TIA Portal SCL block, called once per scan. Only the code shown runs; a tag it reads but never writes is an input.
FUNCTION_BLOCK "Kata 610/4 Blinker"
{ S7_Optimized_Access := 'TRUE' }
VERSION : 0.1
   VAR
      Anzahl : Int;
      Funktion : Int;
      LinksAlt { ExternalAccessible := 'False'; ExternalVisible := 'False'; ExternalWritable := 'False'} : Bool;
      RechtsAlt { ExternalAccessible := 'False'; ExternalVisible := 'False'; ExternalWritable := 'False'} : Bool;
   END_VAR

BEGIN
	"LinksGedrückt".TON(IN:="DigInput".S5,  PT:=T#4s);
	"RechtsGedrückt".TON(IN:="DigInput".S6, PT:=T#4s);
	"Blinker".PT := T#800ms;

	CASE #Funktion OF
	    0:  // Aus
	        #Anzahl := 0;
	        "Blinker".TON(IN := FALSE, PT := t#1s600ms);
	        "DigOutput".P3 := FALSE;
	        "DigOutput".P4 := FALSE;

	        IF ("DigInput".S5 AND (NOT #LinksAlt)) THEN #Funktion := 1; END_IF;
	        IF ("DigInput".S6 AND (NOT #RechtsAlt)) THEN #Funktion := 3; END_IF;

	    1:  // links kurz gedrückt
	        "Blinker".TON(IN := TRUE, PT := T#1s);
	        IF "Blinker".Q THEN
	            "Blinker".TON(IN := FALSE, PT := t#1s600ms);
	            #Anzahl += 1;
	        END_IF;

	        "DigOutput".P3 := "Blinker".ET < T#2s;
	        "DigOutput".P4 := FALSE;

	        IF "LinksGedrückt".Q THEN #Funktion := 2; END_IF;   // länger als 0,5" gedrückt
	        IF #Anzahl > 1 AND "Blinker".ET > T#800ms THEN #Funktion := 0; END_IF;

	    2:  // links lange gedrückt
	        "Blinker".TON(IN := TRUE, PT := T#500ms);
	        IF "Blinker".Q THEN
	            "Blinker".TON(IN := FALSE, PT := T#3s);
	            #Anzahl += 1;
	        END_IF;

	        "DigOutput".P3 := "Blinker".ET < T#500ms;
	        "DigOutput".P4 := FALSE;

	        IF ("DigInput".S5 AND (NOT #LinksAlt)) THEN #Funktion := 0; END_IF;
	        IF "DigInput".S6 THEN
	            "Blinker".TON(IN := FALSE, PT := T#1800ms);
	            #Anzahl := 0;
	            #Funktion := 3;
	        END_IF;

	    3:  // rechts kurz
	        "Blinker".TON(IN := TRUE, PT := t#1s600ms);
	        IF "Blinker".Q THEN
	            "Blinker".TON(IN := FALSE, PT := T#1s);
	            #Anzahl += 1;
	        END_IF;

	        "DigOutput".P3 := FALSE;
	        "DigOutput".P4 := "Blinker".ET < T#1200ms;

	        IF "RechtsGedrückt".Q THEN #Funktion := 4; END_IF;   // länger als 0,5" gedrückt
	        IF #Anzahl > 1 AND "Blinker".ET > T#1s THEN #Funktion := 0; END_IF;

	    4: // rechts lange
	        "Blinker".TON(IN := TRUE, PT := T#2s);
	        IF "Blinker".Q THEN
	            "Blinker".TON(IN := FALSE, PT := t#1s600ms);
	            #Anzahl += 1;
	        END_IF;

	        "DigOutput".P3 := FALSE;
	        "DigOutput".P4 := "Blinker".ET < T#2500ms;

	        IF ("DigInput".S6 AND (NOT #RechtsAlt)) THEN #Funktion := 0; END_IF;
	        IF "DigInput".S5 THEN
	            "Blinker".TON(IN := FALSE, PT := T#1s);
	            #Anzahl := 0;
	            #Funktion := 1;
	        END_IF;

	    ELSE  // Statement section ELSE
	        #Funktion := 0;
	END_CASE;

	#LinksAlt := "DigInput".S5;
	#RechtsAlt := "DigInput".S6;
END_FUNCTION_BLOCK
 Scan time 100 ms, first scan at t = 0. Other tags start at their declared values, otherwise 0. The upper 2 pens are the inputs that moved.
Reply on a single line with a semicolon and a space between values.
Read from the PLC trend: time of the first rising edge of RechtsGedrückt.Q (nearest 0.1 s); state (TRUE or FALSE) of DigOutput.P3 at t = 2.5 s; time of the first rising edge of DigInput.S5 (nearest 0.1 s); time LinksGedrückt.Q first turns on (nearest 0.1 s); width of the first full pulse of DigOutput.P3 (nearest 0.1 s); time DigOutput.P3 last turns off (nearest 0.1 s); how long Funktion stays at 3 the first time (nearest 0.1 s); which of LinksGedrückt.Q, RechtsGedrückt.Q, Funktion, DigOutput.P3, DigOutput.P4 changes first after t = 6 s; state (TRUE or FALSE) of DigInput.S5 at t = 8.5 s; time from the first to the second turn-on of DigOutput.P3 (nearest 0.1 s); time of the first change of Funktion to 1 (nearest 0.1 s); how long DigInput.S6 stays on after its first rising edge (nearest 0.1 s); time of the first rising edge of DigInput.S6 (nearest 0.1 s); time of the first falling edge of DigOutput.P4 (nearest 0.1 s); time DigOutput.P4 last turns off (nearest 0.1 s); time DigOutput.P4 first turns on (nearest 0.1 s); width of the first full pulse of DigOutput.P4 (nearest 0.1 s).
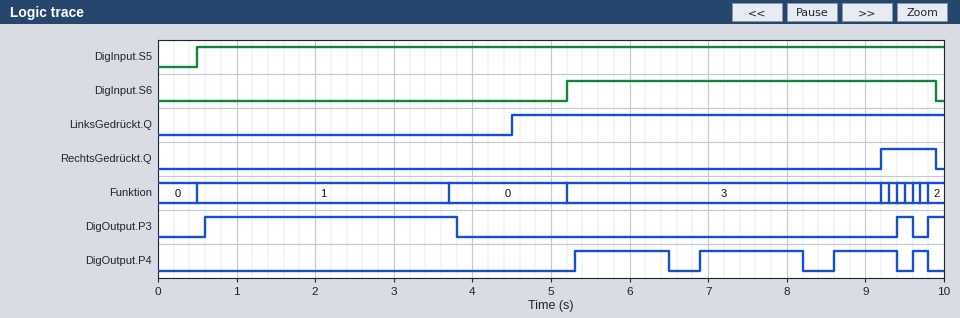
9.2 s; TRUE; 0.5 s; 4.5 s; 3.2 s; 9.6 s; 4.0 s; DigOutput.P4; TRUE; 8.8 s; 0.5 s; 4.7 s; 5.2 s; 6.5 s; 9.8 s; 5.3 s; 1.2 s
